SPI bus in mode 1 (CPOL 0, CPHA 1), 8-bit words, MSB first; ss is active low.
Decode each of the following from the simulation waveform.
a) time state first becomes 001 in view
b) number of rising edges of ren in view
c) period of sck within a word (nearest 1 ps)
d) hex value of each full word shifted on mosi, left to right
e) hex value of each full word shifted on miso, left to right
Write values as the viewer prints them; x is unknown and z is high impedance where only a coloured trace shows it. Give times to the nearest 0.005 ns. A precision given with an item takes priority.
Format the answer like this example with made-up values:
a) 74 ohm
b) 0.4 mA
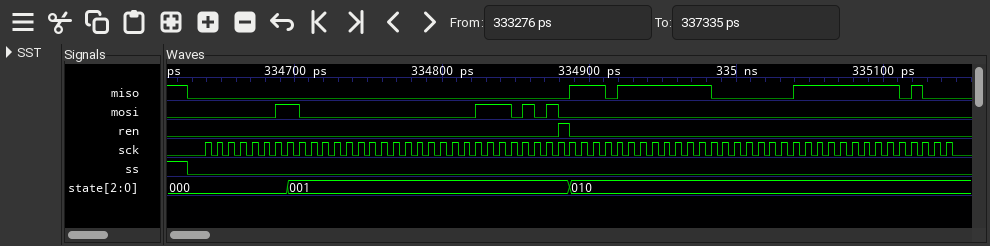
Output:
a) 334.695 ns
b) 1
c) 8 ps
d) 03, 00, 01, D4, 00, 00, 00, 00
e) 00, 00, 00, 01, DF, E0, 3F, E8
